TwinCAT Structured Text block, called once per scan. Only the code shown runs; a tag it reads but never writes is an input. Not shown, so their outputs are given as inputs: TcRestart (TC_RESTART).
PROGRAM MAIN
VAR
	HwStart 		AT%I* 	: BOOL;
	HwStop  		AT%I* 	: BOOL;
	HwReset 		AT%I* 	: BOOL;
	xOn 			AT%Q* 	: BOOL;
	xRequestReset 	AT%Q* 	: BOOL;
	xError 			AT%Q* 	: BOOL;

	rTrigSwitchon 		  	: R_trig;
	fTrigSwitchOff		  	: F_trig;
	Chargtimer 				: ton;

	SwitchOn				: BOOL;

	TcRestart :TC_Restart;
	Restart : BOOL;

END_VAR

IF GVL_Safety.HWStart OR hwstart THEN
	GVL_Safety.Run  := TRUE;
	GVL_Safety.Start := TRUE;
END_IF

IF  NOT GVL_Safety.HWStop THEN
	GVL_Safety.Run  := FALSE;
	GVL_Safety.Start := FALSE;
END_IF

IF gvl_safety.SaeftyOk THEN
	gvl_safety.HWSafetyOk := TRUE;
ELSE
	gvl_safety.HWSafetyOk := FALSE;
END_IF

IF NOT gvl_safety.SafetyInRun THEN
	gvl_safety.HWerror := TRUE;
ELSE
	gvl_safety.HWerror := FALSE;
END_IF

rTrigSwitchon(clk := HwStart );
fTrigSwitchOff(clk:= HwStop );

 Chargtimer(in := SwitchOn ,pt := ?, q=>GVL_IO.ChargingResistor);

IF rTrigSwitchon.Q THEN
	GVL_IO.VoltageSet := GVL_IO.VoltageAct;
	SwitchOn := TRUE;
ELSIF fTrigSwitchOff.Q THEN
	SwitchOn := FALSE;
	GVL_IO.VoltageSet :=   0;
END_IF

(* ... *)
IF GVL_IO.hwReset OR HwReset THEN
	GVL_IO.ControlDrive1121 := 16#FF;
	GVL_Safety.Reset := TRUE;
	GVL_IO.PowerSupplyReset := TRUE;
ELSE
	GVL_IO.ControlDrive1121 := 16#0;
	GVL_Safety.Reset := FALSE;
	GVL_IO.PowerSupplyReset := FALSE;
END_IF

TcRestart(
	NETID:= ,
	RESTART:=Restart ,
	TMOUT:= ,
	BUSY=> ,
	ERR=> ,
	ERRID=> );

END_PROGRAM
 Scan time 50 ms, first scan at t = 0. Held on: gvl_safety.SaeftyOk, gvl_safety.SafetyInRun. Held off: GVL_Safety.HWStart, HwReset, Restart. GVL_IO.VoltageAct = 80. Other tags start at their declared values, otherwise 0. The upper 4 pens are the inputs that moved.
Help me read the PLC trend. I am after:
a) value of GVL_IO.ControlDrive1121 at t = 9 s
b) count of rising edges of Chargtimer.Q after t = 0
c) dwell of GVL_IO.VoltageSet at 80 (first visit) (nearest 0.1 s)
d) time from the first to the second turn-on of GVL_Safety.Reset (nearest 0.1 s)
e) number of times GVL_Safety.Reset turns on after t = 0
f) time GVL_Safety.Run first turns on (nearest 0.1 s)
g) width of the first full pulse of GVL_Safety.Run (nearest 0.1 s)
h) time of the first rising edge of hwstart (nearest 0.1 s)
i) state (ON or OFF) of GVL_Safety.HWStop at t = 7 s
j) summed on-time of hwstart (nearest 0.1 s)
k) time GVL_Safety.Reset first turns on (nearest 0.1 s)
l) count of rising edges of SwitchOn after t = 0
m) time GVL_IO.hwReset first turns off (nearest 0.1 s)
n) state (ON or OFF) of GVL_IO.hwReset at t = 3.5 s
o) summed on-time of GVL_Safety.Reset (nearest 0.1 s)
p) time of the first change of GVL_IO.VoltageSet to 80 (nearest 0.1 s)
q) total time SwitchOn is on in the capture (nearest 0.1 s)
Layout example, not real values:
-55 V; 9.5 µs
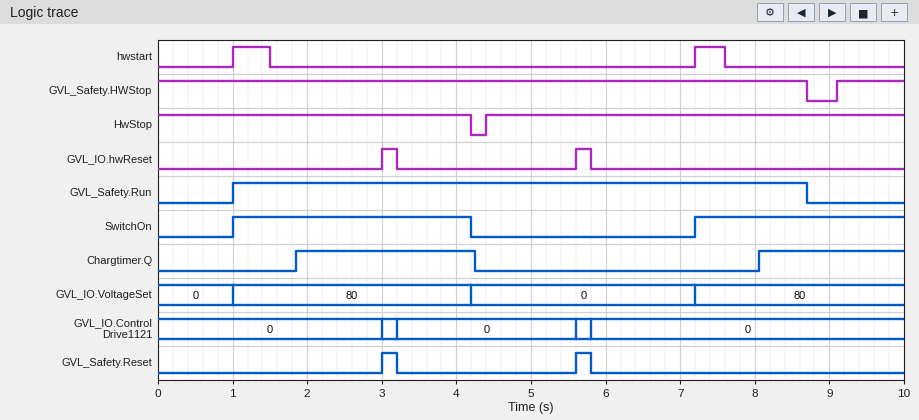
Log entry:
0; 2; 3.2 s; 2.6 s; 2; 1.0 s; 7.7 s; 1.0 s; ON; 0.9 s; 3.0 s; 2; 3.2 s; OFF; 0.4 s; 1.0 s; 6.0 s
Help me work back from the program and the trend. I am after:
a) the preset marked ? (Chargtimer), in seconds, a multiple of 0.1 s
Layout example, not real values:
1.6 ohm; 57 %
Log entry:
0.8 s
